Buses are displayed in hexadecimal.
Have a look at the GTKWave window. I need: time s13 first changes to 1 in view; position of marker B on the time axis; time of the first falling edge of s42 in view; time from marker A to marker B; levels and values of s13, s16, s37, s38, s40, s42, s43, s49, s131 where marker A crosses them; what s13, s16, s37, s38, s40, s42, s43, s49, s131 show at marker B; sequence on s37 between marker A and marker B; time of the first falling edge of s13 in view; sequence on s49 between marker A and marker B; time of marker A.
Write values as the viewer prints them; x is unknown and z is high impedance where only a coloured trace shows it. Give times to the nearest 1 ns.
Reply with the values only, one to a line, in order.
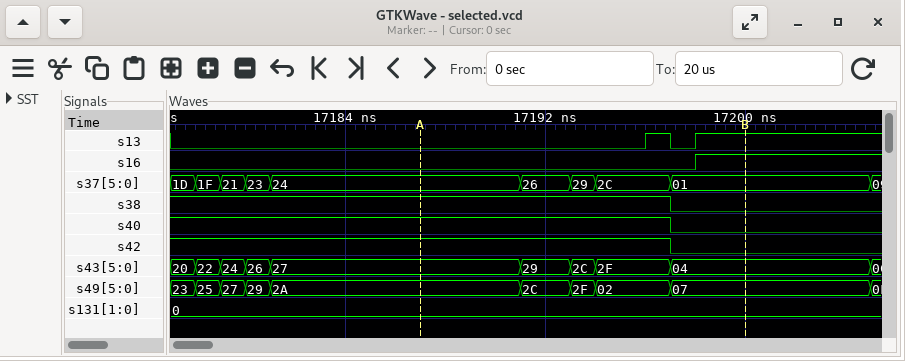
17196 ns
17200 ns
17197 ns
13 ns
s13=0, s16=0, s37=24, s38=1, s40=1, s42=1, s43=27, s49=2A, s131=0
s13=1, s16=1, s37=01, s38=0, s40=0, s42=0, s43=04, s49=07, s131=0
24, 26, 29, 2C, 01
17197 ns
2A, 2C, 2F, 02, 07
17187 ns
